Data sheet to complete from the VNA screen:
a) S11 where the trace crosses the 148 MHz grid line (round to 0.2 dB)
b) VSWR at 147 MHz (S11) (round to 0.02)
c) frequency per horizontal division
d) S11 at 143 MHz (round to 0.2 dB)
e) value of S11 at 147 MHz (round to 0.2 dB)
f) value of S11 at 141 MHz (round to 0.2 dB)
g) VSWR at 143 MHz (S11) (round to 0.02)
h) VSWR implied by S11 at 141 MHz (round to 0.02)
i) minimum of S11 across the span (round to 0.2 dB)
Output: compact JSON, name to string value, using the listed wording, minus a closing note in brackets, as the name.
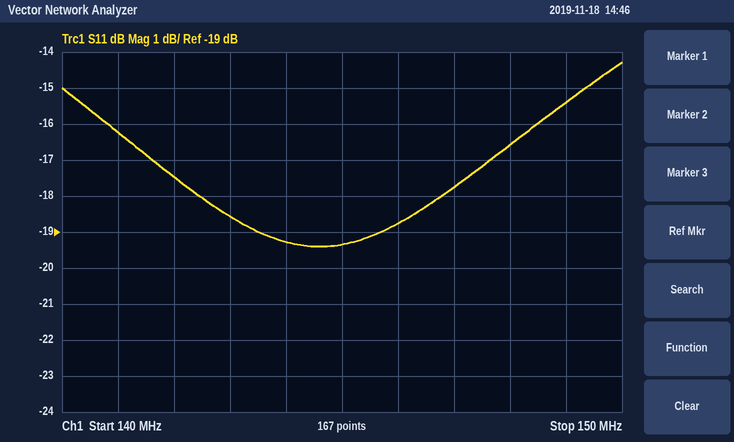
{"S11 where the trace crosses the 148 MHz grid line": "-16.6 dB", "VSWR at 147 MHz (S11)": "1.30", "frequency per horizontal division": "1 MHz", "S11 at 143 MHz": "-18.6 dB", "value of S11 at 147 MHz": "-17.8 dB", "value of S11 at 141 MHz": "-16.2 dB", "VSWR at 143 MHz (S11)": "1.26", "VSWR implied by S11 at 141 MHz": "1.36", "minimum of S11 across the span": "-19.4 dB"}
